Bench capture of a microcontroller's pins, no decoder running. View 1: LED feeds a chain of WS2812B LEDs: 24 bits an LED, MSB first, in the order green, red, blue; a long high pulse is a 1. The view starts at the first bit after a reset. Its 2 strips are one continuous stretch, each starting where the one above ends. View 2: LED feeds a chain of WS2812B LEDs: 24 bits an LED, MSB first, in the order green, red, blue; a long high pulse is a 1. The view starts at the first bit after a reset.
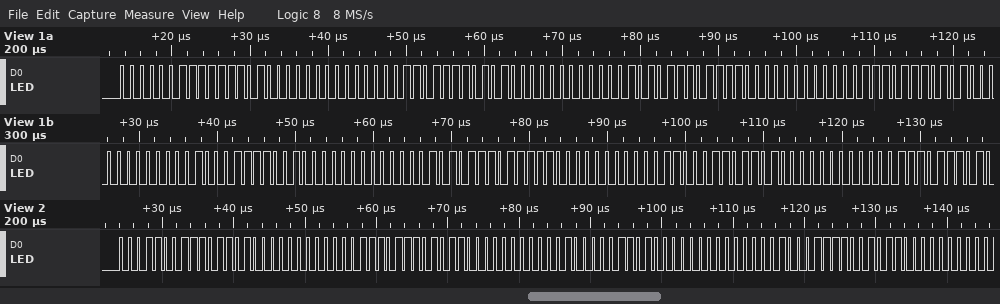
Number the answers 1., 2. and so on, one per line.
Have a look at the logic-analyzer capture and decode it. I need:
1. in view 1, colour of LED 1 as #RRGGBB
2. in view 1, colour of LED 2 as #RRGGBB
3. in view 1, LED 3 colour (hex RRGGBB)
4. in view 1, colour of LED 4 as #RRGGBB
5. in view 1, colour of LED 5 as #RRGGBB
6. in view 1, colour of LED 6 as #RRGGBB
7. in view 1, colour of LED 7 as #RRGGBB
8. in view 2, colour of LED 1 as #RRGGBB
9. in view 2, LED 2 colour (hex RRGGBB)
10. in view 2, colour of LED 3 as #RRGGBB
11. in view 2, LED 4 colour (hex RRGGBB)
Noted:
1. #FA0300
2. #F50600
3. #EF0A00
4. #EA0E00
5. #E41100
6. #DF1500
7. #DA1800
8. #DA1900
9. #D61D00
10. #D02000
11. #CB2300
